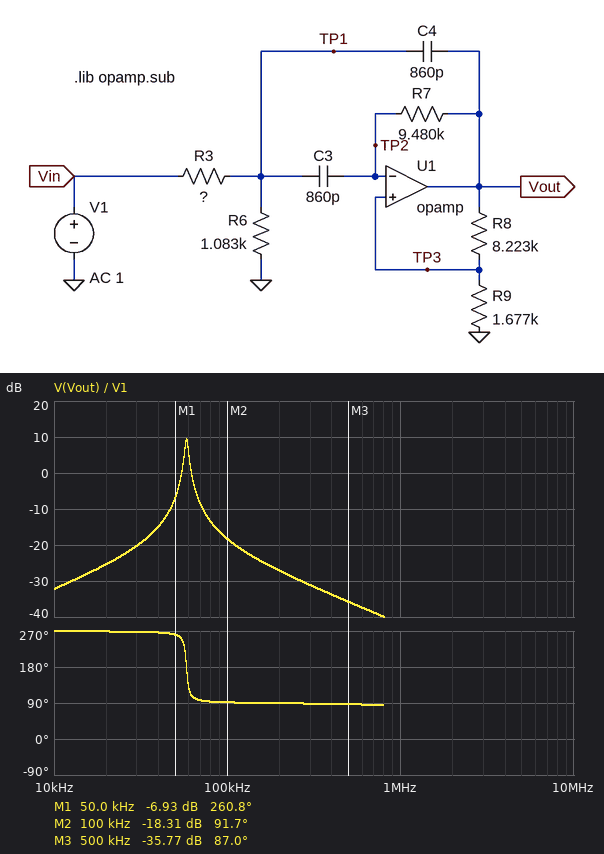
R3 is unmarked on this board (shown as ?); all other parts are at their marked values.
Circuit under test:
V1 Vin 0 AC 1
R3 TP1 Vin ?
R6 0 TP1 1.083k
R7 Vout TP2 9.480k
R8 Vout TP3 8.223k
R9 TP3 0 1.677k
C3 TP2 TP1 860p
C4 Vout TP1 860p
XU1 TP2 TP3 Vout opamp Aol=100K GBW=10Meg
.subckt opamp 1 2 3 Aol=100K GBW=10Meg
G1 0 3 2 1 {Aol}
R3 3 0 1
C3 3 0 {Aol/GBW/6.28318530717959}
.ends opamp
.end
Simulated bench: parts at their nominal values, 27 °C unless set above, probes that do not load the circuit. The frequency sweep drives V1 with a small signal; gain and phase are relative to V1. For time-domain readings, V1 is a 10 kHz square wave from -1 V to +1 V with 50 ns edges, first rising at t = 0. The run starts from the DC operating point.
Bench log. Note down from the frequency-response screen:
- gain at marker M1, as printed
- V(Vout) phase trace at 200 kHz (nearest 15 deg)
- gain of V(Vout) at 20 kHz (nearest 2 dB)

-6.93 dB
90 deg
-26 dB
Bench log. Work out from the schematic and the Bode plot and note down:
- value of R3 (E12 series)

27 kΩ
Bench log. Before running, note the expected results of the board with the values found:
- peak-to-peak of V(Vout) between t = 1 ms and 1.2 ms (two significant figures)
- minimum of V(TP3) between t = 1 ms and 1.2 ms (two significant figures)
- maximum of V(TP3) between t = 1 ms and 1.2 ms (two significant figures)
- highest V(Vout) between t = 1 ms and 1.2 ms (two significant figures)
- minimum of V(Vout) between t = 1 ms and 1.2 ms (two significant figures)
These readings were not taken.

340 mV
-29 mV
29 mV
170 mV
-170 mV
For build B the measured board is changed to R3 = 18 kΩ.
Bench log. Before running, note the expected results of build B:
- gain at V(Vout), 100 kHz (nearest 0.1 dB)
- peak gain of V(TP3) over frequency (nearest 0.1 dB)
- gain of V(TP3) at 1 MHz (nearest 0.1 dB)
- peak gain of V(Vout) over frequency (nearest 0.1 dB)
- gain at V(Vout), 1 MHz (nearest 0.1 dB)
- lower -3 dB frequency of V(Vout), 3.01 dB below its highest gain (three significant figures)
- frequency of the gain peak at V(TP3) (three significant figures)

-14.7 dB
-0.1 dB
-53.8 dB
15.4 dB
-38.4 dB
57.7 kHz
58.7 kHz
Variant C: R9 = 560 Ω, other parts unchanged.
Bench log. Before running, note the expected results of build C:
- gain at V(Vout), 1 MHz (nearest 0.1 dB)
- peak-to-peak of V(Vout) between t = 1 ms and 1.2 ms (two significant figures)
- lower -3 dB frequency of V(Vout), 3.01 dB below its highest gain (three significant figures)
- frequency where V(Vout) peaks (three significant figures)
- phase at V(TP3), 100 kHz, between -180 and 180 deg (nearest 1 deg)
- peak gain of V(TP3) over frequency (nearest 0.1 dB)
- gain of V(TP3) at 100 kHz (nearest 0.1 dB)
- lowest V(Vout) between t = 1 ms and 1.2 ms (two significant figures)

-42.9 dB
360 mV
46.6 kHz
58.3 kHz
111 deg
-35.2 dB
-43.8 dB
-180 mV
